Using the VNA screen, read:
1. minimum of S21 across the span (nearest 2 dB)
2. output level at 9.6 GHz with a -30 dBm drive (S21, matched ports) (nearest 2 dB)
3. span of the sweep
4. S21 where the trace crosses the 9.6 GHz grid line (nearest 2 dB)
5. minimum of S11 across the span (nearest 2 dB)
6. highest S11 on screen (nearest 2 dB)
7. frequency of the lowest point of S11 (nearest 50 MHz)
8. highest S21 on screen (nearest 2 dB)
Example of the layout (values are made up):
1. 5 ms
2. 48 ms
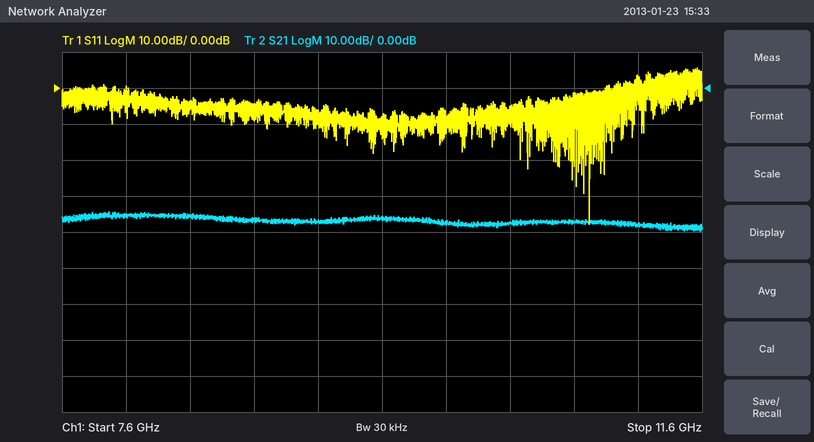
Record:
1. -40 dB
2. -66 dBm
3. 4 GHz
4. -36 dB
5. -38 dB
6. 6 dB
7. 10.90 GHz
8. -34 dB
